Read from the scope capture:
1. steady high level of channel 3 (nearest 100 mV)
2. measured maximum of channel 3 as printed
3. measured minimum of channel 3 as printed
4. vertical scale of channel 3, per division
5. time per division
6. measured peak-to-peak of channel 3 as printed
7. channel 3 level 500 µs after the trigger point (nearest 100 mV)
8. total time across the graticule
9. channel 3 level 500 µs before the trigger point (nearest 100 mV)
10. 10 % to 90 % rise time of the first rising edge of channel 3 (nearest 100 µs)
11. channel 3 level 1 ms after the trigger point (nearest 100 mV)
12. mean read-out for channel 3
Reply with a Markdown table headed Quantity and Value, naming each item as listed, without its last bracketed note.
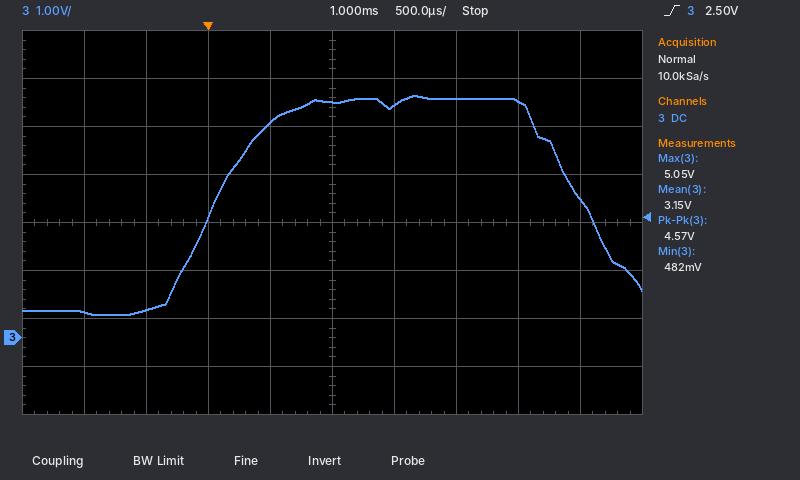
| Quantity | Value |
|---|---|
| steady high level of channel 3 | 5.0 V |
| measured maximum of channel 3 as printed | 5.05 V |
| measured minimum of channel 3 as printed | 482 mV |
| vertical scale of channel 3, per division | 1 V |
| time per division | 500 µs |
| measured peak-to-peak of channel 3 as printed | 4.57 V |
| channel 3 level 500 µs after the trigger point | 4.5 V |
| total time across the graticule | 5 ms |
| channel 3 level 500 µs before the trigger point | 600 mV |
| 10 % to 90 % rise time of the first rising edge of channel 3 | 800 µs |
| channel 3 level 1 ms after the trigger point | 4.9 V |
| mean read-out for channel 3 | 3.15 V |
